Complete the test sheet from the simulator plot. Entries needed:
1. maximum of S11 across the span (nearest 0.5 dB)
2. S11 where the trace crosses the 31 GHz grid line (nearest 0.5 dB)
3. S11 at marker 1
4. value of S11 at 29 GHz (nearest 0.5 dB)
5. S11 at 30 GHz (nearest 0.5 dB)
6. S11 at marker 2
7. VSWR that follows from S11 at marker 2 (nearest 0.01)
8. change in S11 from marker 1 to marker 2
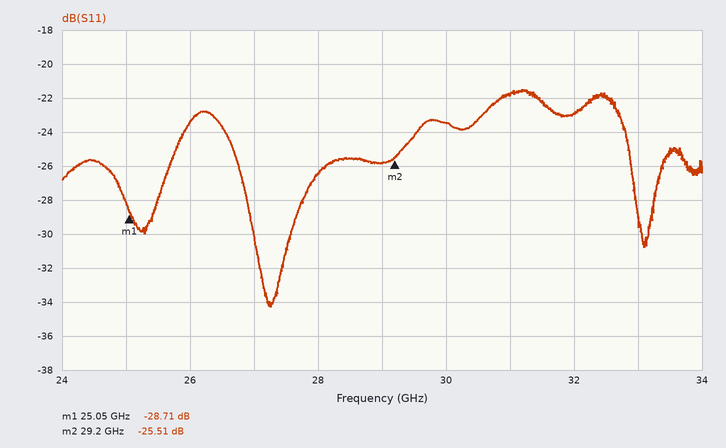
-21.5 dB
-22.0 dB
-28.71 dB
-26.0 dB
-23.5 dB
-25.51 dB
1.11
3.20 dB
